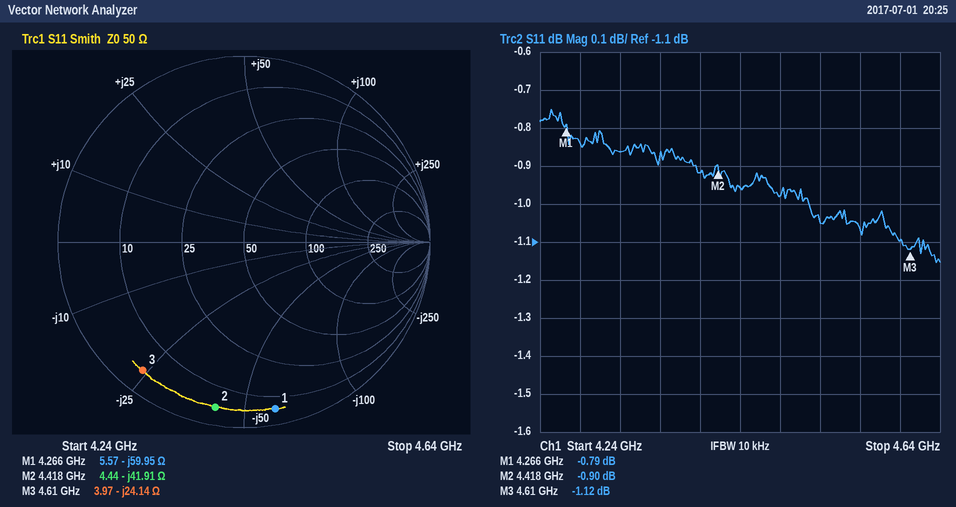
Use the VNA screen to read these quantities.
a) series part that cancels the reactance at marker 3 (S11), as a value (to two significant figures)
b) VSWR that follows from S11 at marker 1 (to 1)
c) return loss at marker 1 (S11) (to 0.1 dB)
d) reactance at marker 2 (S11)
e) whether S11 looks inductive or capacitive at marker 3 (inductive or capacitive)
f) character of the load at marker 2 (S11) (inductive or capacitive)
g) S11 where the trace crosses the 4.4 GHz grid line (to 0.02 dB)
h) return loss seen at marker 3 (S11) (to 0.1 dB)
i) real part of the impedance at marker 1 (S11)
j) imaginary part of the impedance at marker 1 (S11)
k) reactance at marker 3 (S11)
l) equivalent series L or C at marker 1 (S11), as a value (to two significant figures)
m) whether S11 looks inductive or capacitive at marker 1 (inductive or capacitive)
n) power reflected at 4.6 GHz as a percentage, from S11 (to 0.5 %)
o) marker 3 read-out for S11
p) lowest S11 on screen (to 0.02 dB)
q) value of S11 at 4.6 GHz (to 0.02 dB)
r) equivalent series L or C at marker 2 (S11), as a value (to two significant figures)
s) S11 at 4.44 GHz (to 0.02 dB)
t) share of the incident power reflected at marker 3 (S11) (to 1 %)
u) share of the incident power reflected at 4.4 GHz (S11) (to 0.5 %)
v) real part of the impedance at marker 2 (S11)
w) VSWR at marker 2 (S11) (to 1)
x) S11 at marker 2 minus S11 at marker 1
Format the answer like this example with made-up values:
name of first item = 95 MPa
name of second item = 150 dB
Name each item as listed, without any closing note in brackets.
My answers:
series part that cancels the reactance at marker 3 (S11), as a value = 830 pH
VSWR that follows from S11 at marker 1 = 22
return loss at marker 1 (S11) = 0.8 dB
reactance at marker 2 = -41.91 Ω
whether S11 looks inductive or capacitive at marker 3 = capacitive
character of the load at marker 2 (S11) = capacitive
S11 where the trace crosses the 4.4 GHz grid line = -0.92 dB
return loss seen at marker 3 (S11) = 1.1 dB
real part of the impedance at marker 1 = 5.57 Ω
imaginary part of the impedance at marker 1 = -59.95 Ω
reactance at marker 3 = -24.14 Ω
equivalent series L or C at marker 1 (S11), as a value = 620 fF
whether S11 looks inductive or capacitive at marker 1 = capacitive
power reflected at 4.6 GHz as a percentage, from S11 = 77.5 %
marker 3 read-out for S11 = -1.12 dB
lowest S11 on screen = -1.16 dB
value of S11 at 4.6 GHz = -1.10 dB
equivalent series L or C at marker 2 (S11), as a value = 860 fF
S11 at 4.44 GHz = -0.96 dB
share of the incident power reflected at marker 3 (S11) = 77 %
share of the incident power reflected at 4.4 GHz (S11) = 81.0 %
real part of the impedance at marker 2 = 4.44 Ω
VSWR at marker 2 (S11) = 19
S11 at marker 2 minus S11 at marker 1 = -0.11 dB
